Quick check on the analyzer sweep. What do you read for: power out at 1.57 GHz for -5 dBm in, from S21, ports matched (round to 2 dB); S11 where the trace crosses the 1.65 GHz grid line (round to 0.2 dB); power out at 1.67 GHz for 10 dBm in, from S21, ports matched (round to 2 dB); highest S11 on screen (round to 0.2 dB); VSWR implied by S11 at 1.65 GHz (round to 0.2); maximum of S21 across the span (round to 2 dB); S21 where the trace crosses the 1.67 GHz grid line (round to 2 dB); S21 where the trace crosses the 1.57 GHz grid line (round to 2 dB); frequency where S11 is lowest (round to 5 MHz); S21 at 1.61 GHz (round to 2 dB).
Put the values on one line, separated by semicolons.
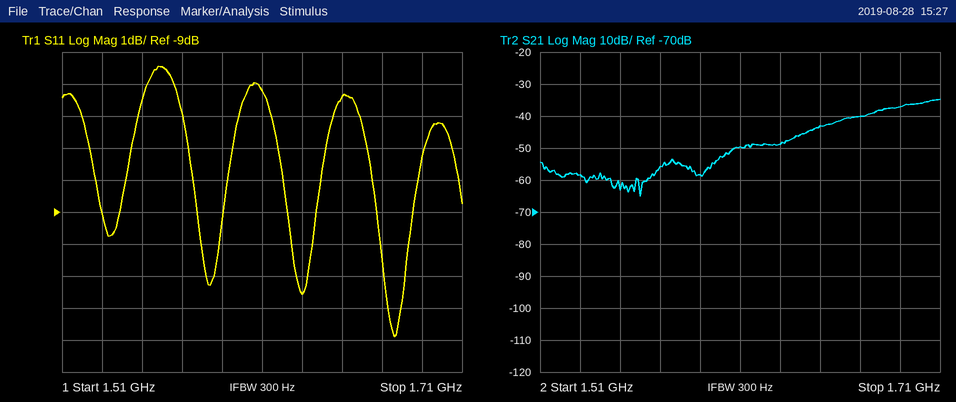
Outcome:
-60 dBm; -5.4 dB; -30 dBm; -4.4 dB; 3.4; -34 dB; -40 dB; -56 dB; 1.675 GHz; -50 dB
